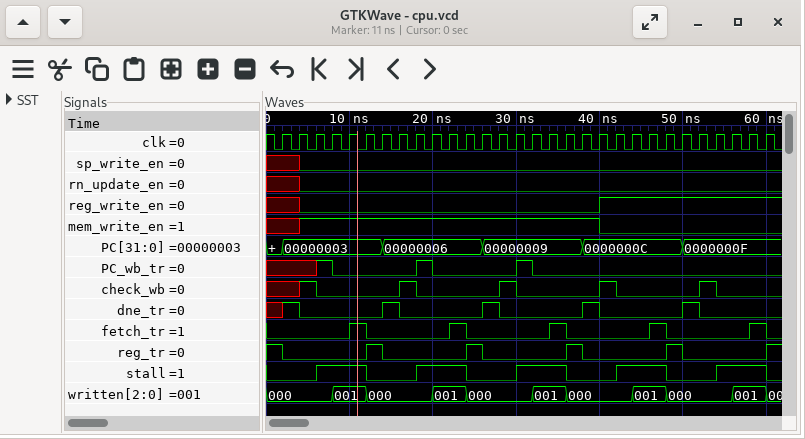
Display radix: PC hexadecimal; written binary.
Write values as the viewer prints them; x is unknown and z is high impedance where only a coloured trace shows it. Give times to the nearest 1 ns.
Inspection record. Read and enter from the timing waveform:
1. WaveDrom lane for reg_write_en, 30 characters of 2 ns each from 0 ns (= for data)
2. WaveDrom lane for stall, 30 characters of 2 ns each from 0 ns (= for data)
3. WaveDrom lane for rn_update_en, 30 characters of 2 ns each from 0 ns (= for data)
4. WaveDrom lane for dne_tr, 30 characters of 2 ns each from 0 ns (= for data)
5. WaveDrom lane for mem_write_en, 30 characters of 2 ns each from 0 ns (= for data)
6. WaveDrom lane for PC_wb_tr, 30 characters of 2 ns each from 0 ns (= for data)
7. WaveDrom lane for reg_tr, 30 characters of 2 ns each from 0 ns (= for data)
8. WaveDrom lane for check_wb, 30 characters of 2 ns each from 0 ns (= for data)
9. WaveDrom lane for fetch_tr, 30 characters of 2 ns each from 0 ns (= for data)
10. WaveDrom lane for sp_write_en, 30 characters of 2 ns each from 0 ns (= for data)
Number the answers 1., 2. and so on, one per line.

1. {name: 'reg_write_en', wave: 'x.0.................1.........'}
2. {name: 'stall', wave: '0..1..0..1..0..1..0..1..0..1..'}
3. {name: 'rn_update_en', wave: 'x.0...........................'}
4. {name: 'dne_tr', wave: 'x10....10....10....10....10...'}
5. {name: 'mem_write_en', wave: 'x.1.................0.........'}
6. {name: 'PC_wb_tr', wave: 'x..10....10....10.............'}
7. {name: 'reg_tr', wave: '10....10....10....10....10....'}
8. {name: 'check_wb', wave: 'x.10....10....10....10....10..'}
9. {name: 'fetch_tr', wave: '0....10....10....10....10....1'}
10. {name: 'sp_write_en', wave: 'x.0...........................'}
